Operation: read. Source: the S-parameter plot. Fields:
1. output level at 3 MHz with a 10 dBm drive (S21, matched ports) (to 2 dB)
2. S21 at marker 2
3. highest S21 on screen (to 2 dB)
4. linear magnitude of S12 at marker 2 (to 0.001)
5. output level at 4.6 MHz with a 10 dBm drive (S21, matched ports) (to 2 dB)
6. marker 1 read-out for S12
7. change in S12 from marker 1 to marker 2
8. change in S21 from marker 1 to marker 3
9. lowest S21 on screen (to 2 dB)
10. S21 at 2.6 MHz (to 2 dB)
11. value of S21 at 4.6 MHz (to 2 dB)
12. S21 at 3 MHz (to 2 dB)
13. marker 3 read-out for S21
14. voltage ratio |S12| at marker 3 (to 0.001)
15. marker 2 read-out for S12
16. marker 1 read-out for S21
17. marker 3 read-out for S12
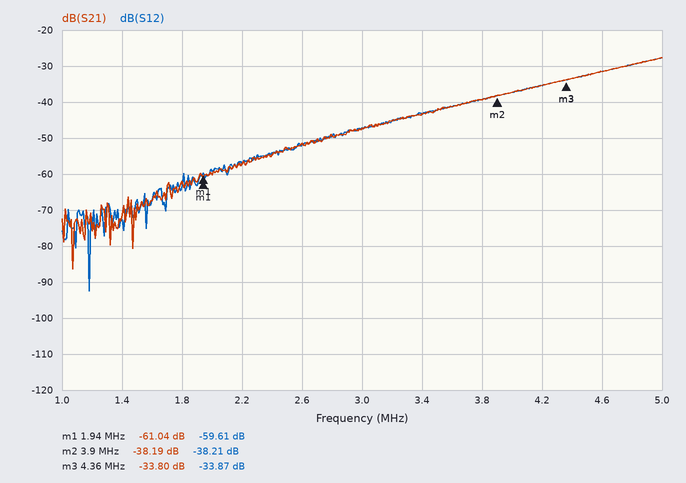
-38 dBm
-38.19 dB
-28 dB
0.012
-22 dBm
-59.61 dB
21.40 dB
27.24 dB
-86 dB
-52 dB
-32 dB
-48 dB
-33.80 dB
0.020
-38.21 dB
-61.04 dB
-33.87 dB
